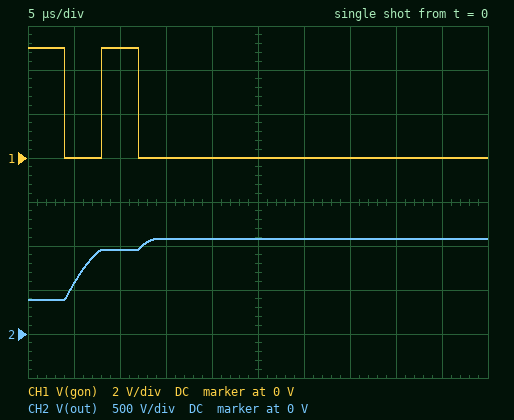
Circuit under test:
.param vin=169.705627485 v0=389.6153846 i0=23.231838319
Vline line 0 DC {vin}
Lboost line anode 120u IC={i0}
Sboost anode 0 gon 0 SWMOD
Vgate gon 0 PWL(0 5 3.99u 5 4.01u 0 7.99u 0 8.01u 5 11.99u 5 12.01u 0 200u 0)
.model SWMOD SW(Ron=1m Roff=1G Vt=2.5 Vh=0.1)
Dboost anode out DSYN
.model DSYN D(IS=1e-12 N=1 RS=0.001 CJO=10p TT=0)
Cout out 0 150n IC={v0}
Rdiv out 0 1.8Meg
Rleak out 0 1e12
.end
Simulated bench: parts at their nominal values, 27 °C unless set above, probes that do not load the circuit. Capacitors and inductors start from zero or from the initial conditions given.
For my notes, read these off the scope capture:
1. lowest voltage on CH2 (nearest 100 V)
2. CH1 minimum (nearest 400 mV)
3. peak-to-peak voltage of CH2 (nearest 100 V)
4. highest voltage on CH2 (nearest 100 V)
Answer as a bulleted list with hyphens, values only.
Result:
- 400 V
- 0 V
- 700 V
- 1.1 kV
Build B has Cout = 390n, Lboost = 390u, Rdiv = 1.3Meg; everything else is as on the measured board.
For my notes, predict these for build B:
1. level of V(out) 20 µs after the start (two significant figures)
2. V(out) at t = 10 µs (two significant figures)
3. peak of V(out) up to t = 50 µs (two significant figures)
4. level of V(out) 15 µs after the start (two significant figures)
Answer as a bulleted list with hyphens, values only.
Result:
- 980 V
- 630 V
- 1.0 kV
- 790 V
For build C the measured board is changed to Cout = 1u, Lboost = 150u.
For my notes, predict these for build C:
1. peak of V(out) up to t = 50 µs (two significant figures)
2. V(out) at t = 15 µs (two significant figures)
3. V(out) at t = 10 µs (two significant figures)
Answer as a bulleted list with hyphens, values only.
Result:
- 610 V
- 550 V
- 490 V
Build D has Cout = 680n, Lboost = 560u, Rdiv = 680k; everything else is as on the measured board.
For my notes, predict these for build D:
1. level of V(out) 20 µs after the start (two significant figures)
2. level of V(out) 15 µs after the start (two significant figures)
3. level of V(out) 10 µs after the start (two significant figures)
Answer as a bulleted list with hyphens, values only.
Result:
- 770 V
- 630 V
- 530 V
